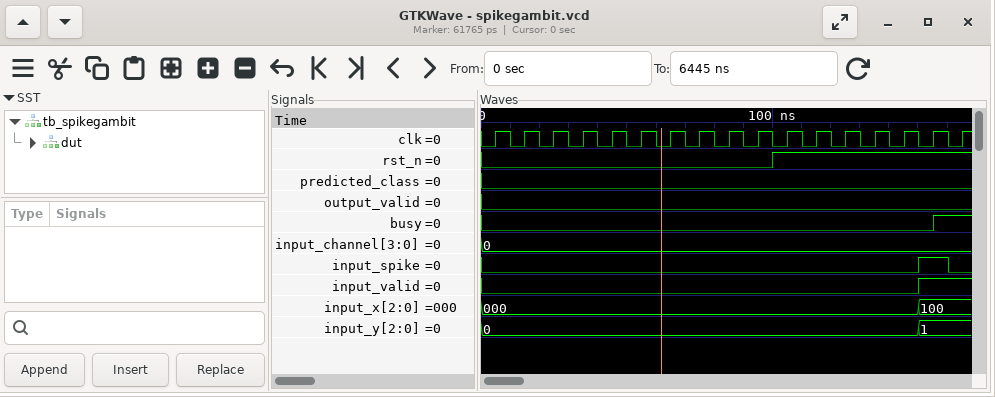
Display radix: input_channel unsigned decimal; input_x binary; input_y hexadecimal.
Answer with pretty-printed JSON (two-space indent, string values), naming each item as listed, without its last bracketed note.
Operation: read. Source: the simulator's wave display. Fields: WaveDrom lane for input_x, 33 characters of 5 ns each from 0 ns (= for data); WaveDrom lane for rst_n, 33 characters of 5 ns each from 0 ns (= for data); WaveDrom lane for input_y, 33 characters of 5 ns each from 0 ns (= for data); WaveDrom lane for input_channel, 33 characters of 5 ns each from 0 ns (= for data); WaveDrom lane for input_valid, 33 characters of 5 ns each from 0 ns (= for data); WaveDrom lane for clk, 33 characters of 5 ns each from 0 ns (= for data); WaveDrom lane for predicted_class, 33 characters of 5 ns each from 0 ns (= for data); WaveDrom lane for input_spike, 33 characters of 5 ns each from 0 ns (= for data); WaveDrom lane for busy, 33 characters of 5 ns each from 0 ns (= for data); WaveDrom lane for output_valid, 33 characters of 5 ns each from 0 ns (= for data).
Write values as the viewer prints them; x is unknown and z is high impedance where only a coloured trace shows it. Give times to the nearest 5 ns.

{
  "WaveDrom lane for input_x, 33 characters of 5 ns each from 0 ns": "{name: 'input_x', wave: '=.............................=..', data: '000 100'}",
  "WaveDrom lane for rst_n, 33 characters of 5 ns each from 0 ns": "{name: 'rst_n', wave: '0...................1............'}",
  "WaveDrom lane for input_y, 33 characters of 5 ns each from 0 ns": "{name: 'input_y', wave: '=.............................=..', data: '0 1'}",
  "WaveDrom lane for input_channel, 33 characters of 5 ns each from 0 ns": "{name: 'input_channel', wave: '=................................', data: '0'}",
  "WaveDrom lane for input_valid, 33 characters of 5 ns each from 0 ns": "{name: 'input_valid', wave: '0.............................1..'}",
  "WaveDrom lane for clk, 33 characters of 5 ns each from 0 ns": "{name: 'clk', wave: '010101010101010101010101010101010'}",
  "WaveDrom lane for predicted_class, 33 characters of 5 ns each from 0 ns": "{name: 'predicted_class', wave: '0................................'}",
  "WaveDrom lane for input_spike, 33 characters of 5 ns each from 0 ns": "{name: 'input_spike', wave: '0.............................1.0'}",
  "WaveDrom lane for busy, 33 characters of 5 ns each from 0 ns": "{name: 'busy', wave: '0..............................1.'}",
  "WaveDrom lane for output_valid, 33 characters of 5 ns each from 0 ns": "{name: 'output_valid', wave: '0................................'}"
}
